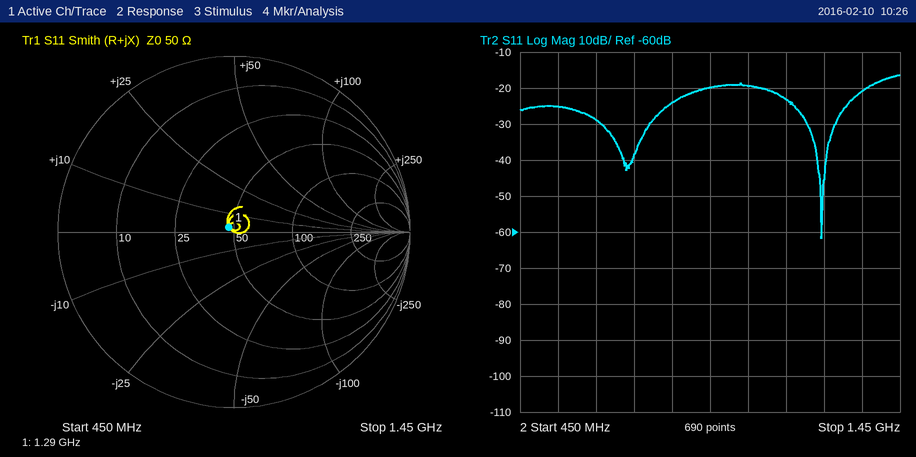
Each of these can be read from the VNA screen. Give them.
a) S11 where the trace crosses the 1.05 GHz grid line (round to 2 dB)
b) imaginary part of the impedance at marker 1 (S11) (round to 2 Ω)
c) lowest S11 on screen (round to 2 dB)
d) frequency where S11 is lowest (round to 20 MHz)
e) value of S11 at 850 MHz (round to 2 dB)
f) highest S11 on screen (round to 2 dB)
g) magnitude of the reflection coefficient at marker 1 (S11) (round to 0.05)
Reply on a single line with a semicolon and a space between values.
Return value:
-20 dB; +2 Ω; -62 dB; 1.24 GHz; -24 dB; -16 dB; 0.05
